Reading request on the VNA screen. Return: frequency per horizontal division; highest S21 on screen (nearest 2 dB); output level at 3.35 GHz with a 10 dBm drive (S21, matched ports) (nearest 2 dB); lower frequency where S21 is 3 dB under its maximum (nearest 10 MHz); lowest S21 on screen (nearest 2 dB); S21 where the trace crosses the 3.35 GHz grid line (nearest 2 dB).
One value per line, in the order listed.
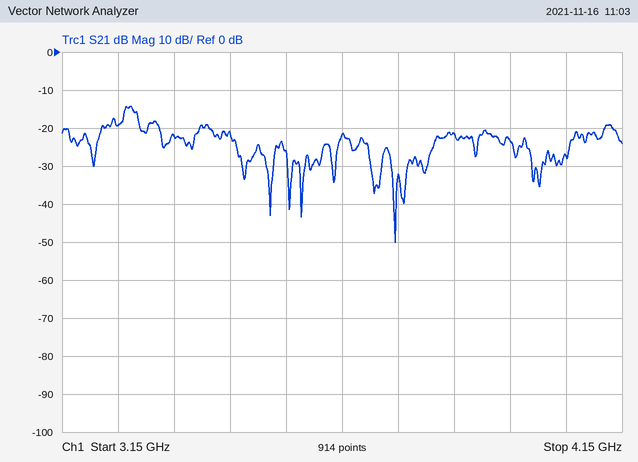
100 MHz
-14 dB
-12 dBm
3.26 GHz
-50 dB
-22 dB
